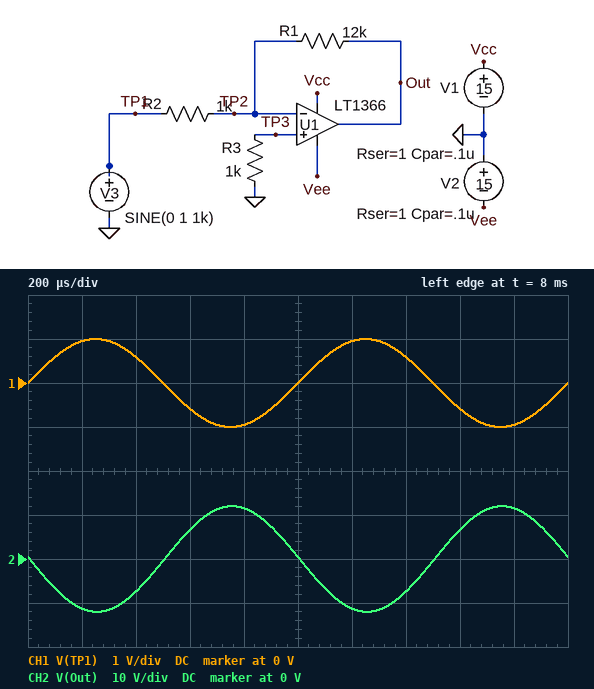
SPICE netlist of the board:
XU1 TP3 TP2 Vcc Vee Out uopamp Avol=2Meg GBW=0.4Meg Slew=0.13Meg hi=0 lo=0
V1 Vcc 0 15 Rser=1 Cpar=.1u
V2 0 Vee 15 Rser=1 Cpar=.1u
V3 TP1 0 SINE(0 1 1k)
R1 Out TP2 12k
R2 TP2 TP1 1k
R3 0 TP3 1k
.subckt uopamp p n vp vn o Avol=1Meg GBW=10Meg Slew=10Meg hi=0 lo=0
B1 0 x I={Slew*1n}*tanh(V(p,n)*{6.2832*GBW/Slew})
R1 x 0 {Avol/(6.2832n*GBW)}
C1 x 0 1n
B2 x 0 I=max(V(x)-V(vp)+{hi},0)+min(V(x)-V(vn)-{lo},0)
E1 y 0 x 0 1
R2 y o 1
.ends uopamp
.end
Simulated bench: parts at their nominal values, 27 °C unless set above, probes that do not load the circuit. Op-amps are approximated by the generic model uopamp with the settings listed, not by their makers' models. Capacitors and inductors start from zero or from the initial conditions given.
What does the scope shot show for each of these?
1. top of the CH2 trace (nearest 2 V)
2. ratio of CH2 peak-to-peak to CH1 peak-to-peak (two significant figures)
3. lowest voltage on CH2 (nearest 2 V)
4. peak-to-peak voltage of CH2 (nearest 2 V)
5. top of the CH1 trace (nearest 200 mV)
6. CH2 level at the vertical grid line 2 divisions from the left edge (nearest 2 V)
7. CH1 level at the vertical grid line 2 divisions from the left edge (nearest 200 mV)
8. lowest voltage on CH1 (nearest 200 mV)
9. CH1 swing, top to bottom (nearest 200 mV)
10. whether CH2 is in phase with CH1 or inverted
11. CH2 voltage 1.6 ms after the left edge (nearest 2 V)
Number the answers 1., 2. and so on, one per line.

1. 12 V
2. 12
3. -12 V
4. 24 V
5. 1.0 V
6. -8 V
7. 600 mV
8. -1.0 V
9. 2.0 V
10. inverted
11. 6 V
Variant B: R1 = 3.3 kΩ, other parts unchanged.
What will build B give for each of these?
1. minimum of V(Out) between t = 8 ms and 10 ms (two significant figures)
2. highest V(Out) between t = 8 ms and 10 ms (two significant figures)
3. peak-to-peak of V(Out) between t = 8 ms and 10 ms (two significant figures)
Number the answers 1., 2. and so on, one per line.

1. -3.3 V
2. 3.3 V
3. 6.6 V
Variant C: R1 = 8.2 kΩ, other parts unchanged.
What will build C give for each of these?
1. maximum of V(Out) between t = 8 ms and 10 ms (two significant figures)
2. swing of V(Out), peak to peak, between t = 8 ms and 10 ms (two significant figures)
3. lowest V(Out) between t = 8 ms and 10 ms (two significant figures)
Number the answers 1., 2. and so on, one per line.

1. 8.2 V
2. 16 V
3. -8.2 V
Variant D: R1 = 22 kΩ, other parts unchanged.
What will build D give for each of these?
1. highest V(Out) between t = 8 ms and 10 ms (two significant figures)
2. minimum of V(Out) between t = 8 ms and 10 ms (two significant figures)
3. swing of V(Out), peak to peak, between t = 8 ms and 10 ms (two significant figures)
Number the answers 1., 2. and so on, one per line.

1. 15 V
2. -15 V
3. 30 V
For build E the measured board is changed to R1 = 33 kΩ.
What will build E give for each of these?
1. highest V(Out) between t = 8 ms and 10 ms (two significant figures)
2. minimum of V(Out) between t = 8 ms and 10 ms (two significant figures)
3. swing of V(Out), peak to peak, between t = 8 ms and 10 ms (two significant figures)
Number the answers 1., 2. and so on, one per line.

1. 15 V
2. -15 V
3. 30 V
